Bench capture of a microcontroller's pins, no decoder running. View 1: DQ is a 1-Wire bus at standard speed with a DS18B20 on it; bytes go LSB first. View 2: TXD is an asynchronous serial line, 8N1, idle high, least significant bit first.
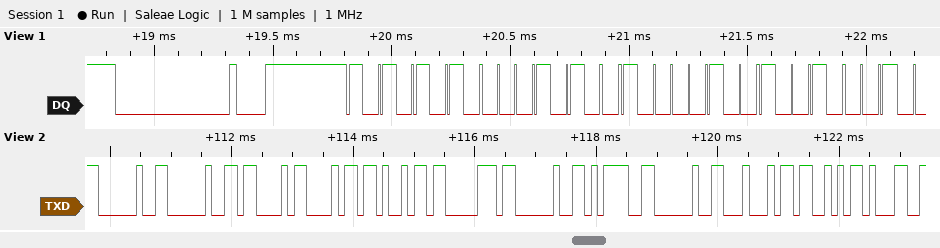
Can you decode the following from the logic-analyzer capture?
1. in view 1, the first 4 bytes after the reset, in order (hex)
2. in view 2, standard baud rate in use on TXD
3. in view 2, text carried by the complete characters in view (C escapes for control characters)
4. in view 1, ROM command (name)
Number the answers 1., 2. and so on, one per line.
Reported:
1. 55 28 21 89
2. 9600 baud
3. "  Chip = DS1"
4. Match ROM
